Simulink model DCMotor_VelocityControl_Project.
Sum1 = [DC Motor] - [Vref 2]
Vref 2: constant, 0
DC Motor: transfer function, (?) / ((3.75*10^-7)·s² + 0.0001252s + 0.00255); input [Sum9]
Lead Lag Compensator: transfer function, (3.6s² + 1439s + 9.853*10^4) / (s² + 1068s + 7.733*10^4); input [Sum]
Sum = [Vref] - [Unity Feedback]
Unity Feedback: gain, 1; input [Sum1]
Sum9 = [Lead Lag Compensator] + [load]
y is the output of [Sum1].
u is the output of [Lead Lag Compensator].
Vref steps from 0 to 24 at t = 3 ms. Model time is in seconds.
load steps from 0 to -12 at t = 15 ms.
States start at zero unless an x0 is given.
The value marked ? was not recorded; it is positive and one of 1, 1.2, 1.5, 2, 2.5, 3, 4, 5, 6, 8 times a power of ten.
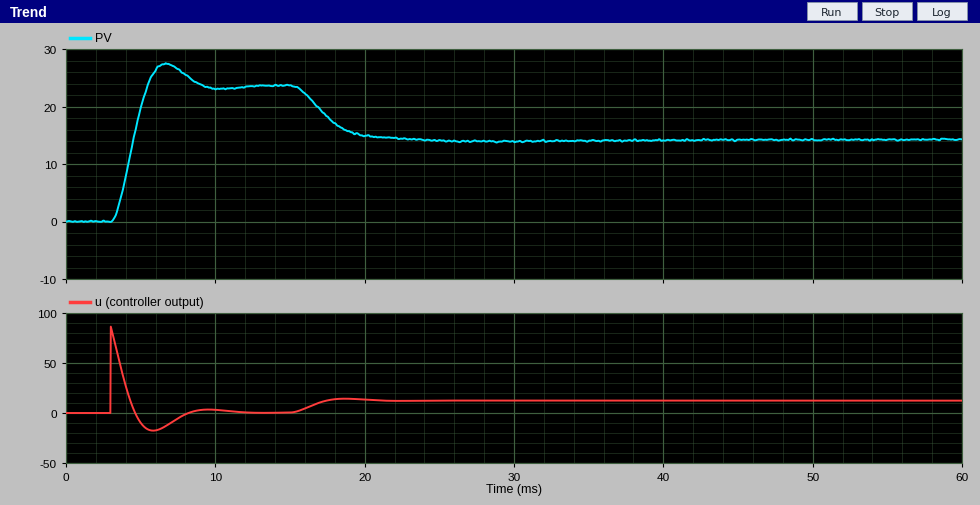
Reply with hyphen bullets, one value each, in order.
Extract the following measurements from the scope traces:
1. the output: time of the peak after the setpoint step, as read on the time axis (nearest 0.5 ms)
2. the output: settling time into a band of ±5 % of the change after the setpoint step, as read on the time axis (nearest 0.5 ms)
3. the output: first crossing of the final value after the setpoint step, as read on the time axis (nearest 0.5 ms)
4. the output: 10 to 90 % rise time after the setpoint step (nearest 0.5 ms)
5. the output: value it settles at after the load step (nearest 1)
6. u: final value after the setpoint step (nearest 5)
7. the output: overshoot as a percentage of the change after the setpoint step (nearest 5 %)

- 6.5 ms
- 8.5 ms
- 5.5 ms
- 1.5 ms
- 14
- 0
- 15 %
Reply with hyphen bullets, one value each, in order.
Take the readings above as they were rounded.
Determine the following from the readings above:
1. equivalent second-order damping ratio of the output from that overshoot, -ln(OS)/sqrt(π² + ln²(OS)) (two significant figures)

- 0.52
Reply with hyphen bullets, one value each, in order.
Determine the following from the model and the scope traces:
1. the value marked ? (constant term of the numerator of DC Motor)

- 0.1
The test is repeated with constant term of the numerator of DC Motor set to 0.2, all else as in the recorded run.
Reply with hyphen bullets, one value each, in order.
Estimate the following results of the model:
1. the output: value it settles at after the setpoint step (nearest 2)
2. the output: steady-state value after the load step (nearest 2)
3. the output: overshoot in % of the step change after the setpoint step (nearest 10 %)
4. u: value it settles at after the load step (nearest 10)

- 24
- 14
- 30 %
- 10
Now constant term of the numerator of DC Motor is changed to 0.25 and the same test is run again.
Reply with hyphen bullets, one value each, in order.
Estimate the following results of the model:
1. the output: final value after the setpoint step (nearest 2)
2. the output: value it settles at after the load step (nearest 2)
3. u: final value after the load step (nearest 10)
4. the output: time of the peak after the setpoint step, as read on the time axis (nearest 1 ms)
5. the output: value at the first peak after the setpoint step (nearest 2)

- 24
- 14
- 10
- 5 ms
- 32
